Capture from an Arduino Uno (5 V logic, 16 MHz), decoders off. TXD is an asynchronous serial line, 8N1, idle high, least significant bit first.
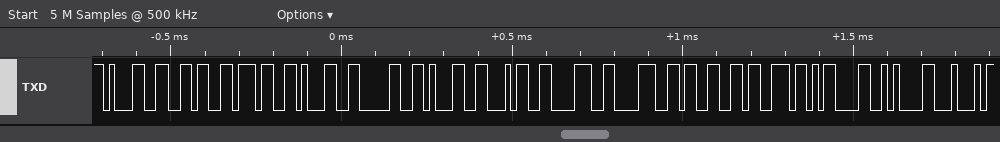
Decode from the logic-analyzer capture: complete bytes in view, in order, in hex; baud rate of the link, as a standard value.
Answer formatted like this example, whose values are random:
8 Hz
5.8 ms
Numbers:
0x31 0x36 0x37 0x31 0x30 0x31 0x34 0x38 0x38 0x33 0x73 0x0D 0x0A 0x44
57600 baud
